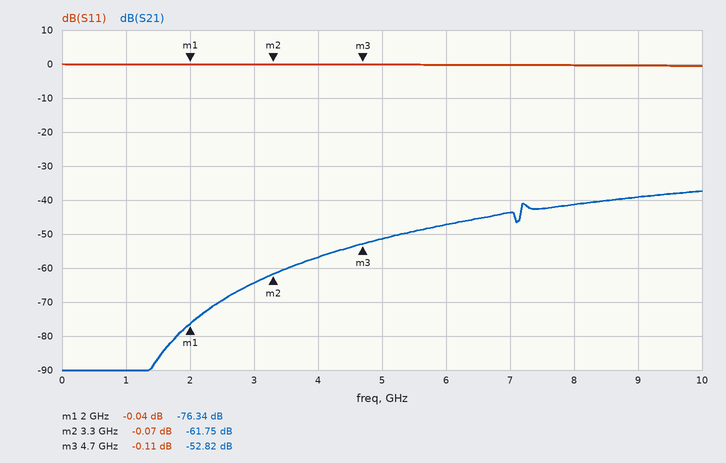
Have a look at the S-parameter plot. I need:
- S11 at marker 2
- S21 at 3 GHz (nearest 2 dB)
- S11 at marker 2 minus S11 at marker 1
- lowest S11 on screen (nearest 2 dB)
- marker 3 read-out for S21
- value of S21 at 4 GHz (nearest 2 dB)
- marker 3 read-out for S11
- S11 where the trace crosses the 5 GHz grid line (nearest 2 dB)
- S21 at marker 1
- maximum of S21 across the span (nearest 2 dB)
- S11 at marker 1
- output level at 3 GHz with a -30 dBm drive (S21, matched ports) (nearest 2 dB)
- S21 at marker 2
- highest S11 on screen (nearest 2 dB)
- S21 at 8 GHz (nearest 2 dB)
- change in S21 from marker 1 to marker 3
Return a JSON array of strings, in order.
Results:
["-0.07 dB", "-64 dB", "-0.03 dB", "0 dB", "-52.82 dB", "-56 dB", "-0.11 dB", "0 dB", "-76.34 dB", "-38 dB", "-0.04 dB", "-94 dBm", "-61.75 dB", "0 dB", "-42 dB", "23.52 dB"]
